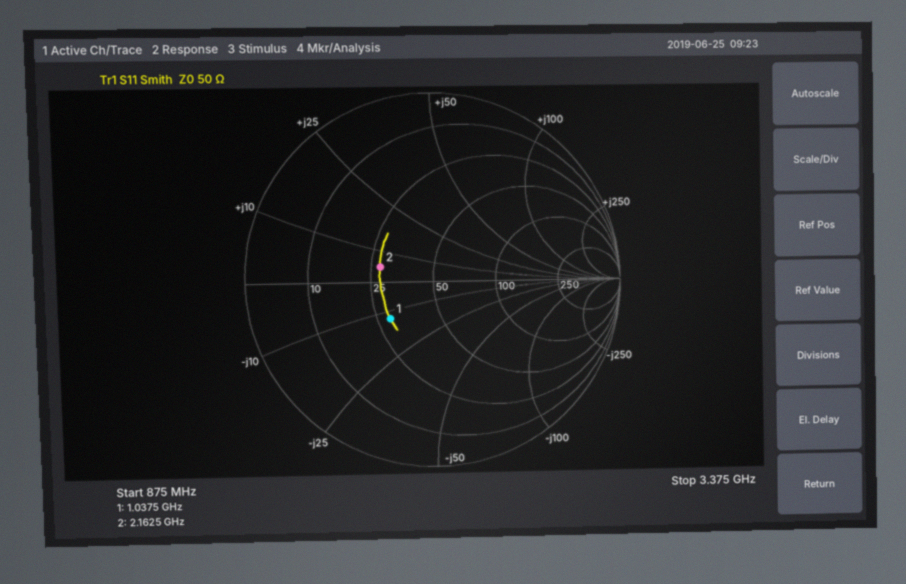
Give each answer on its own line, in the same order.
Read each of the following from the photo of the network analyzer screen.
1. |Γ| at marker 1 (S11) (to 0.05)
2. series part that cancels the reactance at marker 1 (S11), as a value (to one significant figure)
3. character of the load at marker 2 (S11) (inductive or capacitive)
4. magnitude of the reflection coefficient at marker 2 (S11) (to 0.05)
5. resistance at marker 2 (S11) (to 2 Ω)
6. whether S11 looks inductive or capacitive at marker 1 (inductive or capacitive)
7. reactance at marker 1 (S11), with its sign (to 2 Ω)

0.30
2 nH
inductive
0.30
28 Ω
capacitive
-12 Ω
